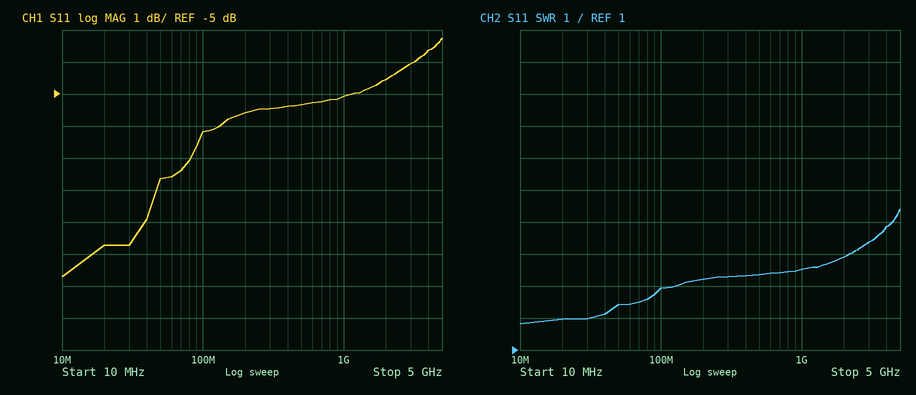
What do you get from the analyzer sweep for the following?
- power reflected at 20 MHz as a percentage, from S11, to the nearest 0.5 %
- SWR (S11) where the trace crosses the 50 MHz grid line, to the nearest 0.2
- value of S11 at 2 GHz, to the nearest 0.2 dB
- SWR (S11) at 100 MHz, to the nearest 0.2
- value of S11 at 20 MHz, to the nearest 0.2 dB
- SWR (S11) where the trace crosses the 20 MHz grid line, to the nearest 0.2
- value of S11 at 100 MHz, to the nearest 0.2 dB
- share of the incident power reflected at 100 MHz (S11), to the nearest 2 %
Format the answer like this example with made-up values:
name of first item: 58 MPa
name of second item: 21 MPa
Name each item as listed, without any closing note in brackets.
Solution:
power reflected at 20 MHz as a percentage, from S11, to the nearest 0.5 %: 10.5 %
SWR (S11) where the trace crosses the 50 MHz grid line, to the nearest 0.2: 2.4
value of S11 at 2 GHz, to the nearest 0.2 dB: -4.6 dB
SWR (S11) at 100 MHz, to the nearest 0.2: 3.0
value of S11 at 20 MHz, to the nearest 0.2 dB: -9.8 dB
SWR (S11) where the trace crosses the 20 MHz grid line, to the nearest 0.2: 2.0
value of S11 at 100 MHz, to the nearest 0.2 dB: -6.2 dB
share of the incident power reflected at 100 MHz (S11), to the nearest 2 %: 24 %
